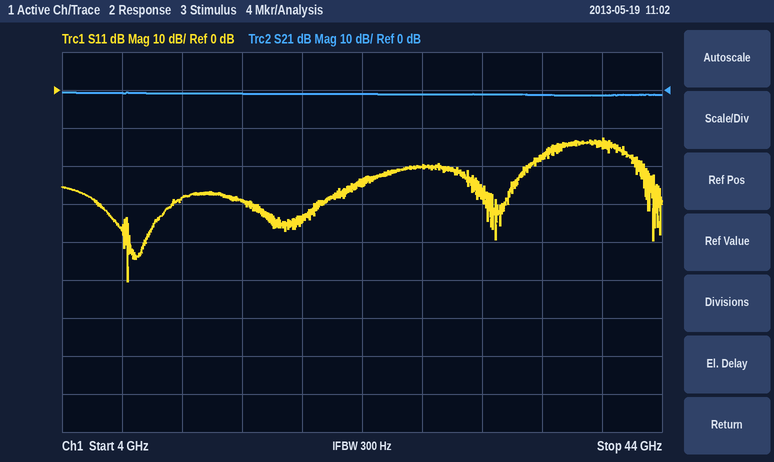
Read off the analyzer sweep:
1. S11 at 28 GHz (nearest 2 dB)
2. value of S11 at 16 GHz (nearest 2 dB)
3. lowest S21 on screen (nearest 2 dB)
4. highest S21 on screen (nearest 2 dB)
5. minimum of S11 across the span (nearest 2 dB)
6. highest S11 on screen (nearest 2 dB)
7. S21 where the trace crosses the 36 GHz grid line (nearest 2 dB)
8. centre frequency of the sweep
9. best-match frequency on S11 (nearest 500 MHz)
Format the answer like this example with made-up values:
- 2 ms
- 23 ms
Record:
- -20 dB
- -30 dB
- -2 dB
- 0 dB
- -50 dB
- -12 dB
- -2 dB
- 24 GHz
- 8.5 GHz
